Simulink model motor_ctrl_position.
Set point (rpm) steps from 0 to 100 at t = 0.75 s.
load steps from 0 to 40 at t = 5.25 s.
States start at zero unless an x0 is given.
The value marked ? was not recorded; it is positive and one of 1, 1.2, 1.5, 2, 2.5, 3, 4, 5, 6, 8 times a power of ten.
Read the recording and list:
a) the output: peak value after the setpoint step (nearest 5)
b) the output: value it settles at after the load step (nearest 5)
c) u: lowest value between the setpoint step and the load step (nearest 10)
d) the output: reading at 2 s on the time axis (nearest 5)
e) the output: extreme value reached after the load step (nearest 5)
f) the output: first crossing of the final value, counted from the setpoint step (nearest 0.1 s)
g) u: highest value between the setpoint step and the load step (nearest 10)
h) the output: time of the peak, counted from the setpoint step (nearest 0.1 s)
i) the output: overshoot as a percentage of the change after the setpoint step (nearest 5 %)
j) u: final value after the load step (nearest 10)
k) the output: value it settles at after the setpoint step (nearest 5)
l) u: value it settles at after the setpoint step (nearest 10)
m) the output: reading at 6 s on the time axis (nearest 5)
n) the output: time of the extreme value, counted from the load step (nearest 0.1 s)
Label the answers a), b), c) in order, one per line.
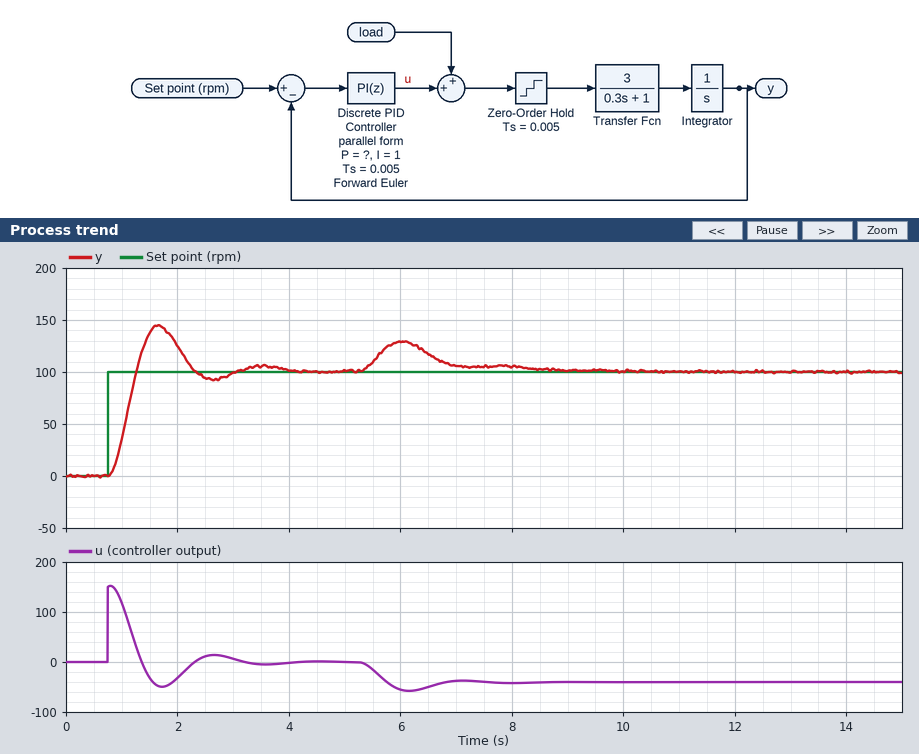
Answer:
a) 145
b) 100
c) -50
d) 125
e) 130
f) 0.5 s
g) 150
h) 0.9 s
i) 45 %
j) -40
k) 100
l) 0
m) 130
n) 0.8 s
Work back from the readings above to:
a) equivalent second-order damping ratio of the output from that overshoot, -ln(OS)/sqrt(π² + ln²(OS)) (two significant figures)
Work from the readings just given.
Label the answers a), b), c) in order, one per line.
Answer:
a) 0.25
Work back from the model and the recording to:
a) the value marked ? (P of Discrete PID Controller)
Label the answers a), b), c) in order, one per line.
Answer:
a) 1.5
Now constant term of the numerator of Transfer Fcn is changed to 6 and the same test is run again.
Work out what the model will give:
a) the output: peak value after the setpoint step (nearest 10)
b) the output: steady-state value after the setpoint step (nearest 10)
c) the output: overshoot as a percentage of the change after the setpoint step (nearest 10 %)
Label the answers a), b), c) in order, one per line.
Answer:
a) 150
b) 100
c) 50 %
